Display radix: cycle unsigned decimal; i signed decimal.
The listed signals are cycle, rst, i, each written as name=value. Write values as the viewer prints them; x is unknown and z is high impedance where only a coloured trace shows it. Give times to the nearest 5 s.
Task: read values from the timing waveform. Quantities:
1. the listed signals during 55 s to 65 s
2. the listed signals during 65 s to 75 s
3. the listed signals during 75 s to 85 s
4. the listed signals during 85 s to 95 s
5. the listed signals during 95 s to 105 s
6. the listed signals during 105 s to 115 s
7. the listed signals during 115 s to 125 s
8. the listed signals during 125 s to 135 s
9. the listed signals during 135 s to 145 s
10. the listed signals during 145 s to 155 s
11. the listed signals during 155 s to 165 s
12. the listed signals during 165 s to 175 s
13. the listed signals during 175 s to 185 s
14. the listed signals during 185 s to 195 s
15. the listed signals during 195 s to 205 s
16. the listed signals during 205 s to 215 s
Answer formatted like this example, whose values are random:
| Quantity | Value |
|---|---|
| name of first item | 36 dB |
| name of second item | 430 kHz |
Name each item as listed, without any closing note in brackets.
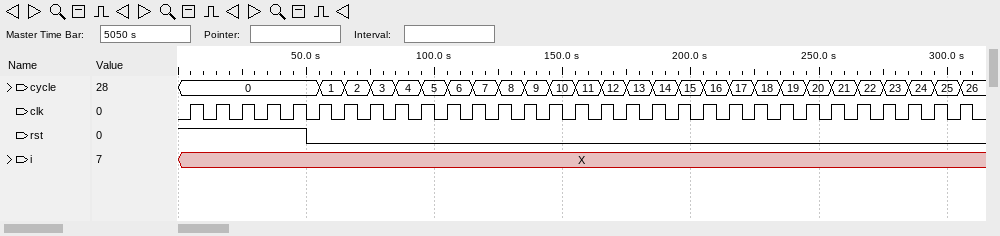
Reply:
| Quantity | Value |
|---|---|
| the listed signals during 55 s to 65 s | cycle=1, rst=0, i=X |
| the listed signals during 65 s to 75 s | cycle=2, rst=0, i=X |
| the listed signals during 75 s to 85 s | cycle=3, rst=0, i=X |
| the listed signals during 85 s to 95 s | cycle=4, rst=0, i=X |
| the listed signals during 95 s to 105 s | cycle=5, rst=0, i=X |
| the listed signals during 105 s to 115 s | cycle=6, rst=0, i=X |
| the listed signals during 115 s to 125 s | cycle=7, rst=0, i=X |
| the listed signals during 125 s to 135 s | cycle=8, rst=0, i=X |
| the listed signals during 135 s to 145 s | cycle=9, rst=0, i=X |
| the listed signals during 145 s to 155 s | cycle=10, rst=0, i=X |
| the listed signals during 155 s to 165 s | cycle=11, rst=0, i=X |
| the listed signals during 165 s to 175 s | cycle=12, rst=0, i=X |
| the listed signals during 175 s to 185 s | cycle=13, rst=0, i=X |
| the listed signals during 185 s to 195 s | cycle=14, rst=0, i=X |
| the listed signals during 195 s to 205 s | cycle=15, rst=0, i=X |
| the listed signals during 205 s to 215 s | cycle=16, rst=0, i=X |
